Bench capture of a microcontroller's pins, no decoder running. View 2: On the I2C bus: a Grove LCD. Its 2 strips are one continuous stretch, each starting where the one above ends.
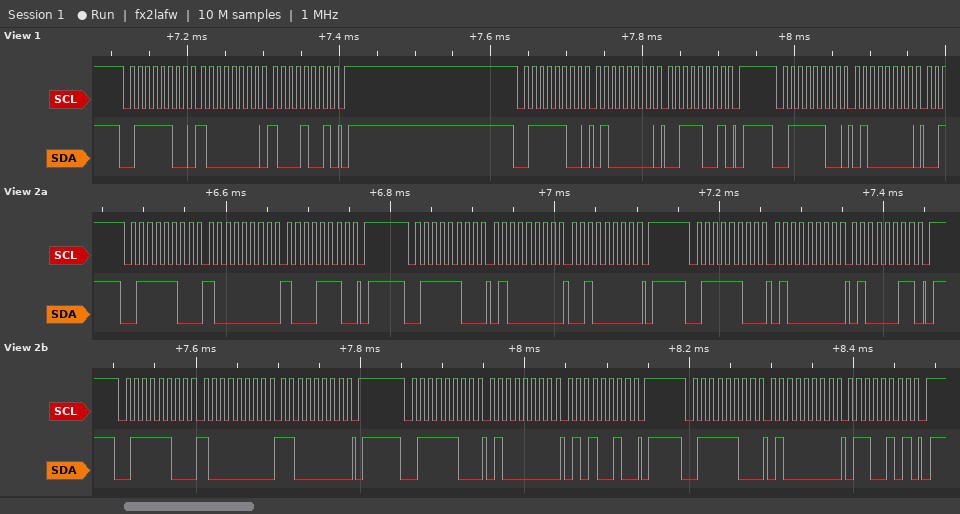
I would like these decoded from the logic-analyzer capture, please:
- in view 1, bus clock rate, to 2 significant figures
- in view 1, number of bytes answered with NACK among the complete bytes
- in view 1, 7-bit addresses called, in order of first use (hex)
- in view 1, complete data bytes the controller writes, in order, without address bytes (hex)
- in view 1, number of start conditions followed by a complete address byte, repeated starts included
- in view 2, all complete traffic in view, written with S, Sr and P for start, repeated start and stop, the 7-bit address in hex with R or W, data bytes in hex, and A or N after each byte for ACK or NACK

100 kHz
0
0x3E
80 89 40 39 40
3
S 3EW A 80 A 8E A P S 3EW A 40 A 20 A P S 3EW A 40 A 43 A P S 3EW A 80 A C0 A P S 3EW A 40 A 52 A P S 3EW A 40 A 65 A P
